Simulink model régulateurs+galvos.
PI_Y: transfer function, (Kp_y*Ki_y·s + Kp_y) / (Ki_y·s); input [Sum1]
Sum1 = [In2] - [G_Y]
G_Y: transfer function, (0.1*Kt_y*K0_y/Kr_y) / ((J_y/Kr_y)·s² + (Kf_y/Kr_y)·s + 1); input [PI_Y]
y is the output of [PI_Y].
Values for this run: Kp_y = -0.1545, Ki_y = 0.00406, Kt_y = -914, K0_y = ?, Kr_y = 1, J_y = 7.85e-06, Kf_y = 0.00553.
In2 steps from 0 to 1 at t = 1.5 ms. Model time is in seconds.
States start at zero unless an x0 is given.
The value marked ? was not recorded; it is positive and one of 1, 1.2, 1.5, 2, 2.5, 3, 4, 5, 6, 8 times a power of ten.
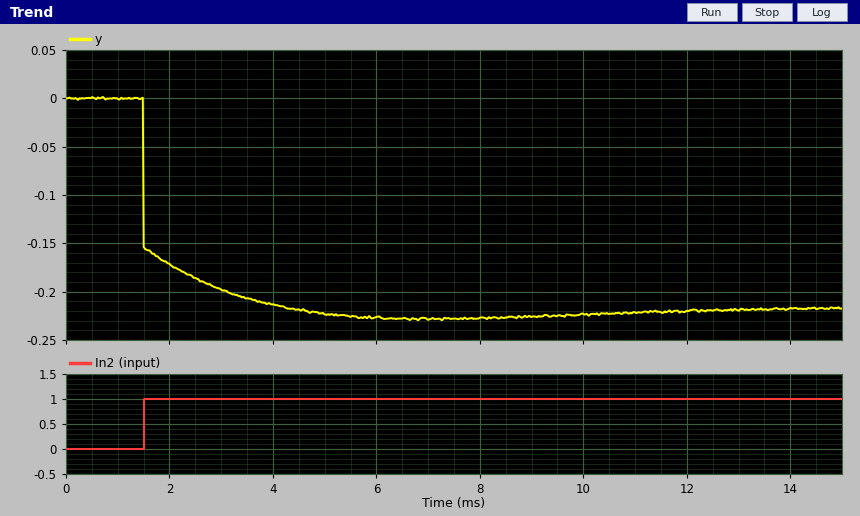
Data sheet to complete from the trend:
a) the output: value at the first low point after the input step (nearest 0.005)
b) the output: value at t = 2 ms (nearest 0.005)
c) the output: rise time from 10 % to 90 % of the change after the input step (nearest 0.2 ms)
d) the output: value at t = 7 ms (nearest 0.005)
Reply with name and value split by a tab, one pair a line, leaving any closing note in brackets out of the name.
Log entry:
the output: value at the first low point after the input step	-0.230
the output: value at t = 2 ms	-0.170
the output: rise time from 10 % to 90 % of the change after the input step	1.4 ms
the output: value at t = 7 ms	-0.230
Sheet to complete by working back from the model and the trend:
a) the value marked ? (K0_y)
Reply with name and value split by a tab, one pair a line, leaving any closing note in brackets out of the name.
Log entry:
the value marked ?	0.05
